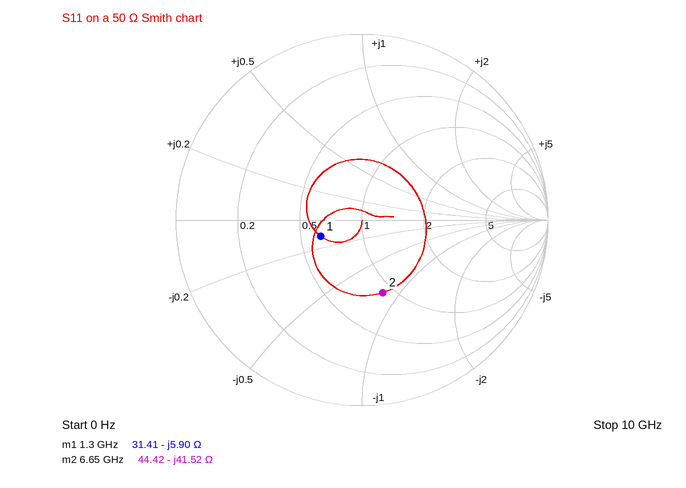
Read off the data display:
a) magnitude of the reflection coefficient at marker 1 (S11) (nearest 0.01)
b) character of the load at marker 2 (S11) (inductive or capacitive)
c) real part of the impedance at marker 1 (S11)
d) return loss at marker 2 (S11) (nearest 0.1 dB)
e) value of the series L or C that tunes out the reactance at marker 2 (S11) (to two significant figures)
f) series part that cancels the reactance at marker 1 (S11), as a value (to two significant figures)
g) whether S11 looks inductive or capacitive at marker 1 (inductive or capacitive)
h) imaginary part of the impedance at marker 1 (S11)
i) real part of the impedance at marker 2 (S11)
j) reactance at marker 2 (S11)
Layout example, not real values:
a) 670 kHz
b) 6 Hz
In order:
a) 0.24
b) capacitive
c) 31.41 Ω
d) 7.8 dB
e) 990 pH
f) 720 pH
g) capacitive
h) -5.90 Ω
i) 44.42 Ω
j) -41.52 Ω
